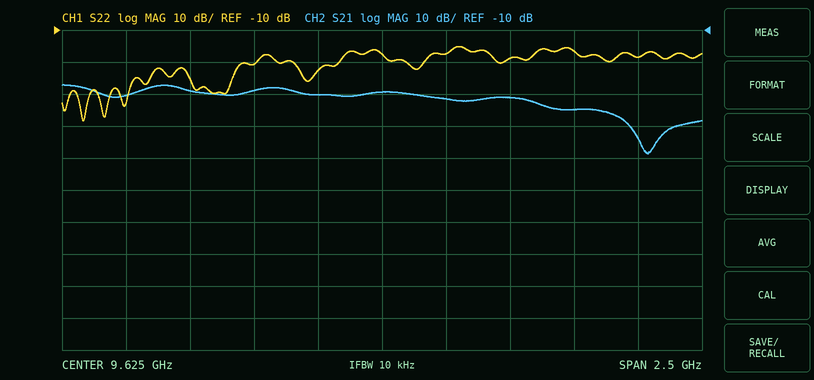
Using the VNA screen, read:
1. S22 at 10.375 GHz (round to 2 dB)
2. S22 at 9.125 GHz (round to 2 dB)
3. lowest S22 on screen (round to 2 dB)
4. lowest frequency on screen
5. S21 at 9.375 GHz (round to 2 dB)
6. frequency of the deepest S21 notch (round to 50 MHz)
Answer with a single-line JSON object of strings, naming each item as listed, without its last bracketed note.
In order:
{"S22 at 10.375 GHz": "-16 dB", "S22 at 9.125 GHz": "-20 dB", "lowest S22 on screen": "-38 dB", "lowest frequency on screen": "8.375 GHz", "S21 at 9.375 GHz": "-30 dB", "frequency of the deepest S21 notch": "10.65 GHz"}
